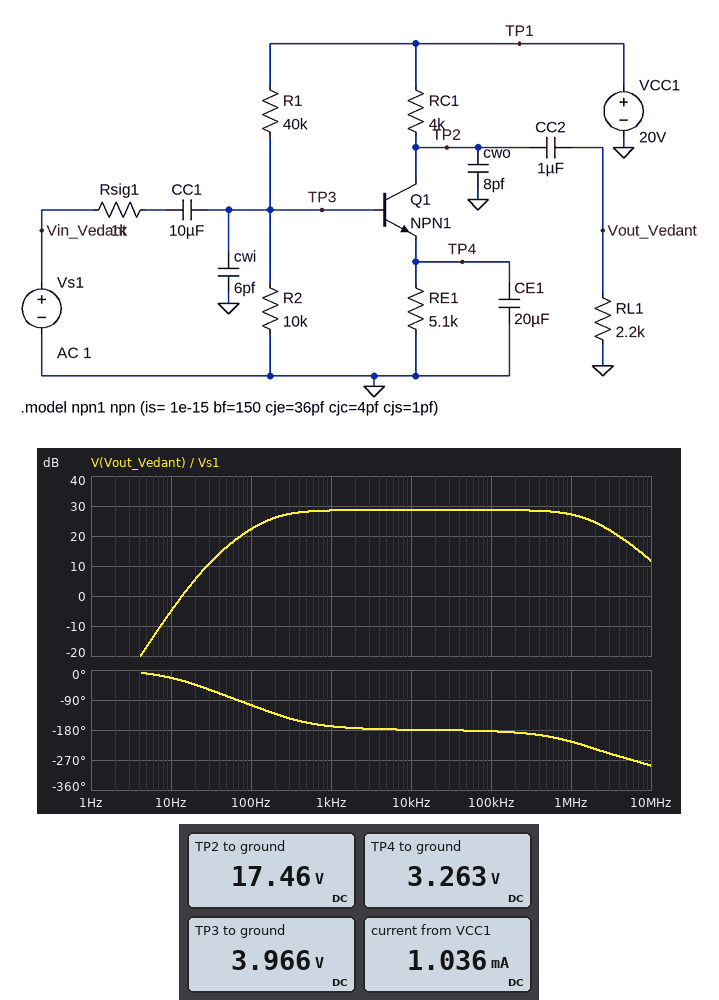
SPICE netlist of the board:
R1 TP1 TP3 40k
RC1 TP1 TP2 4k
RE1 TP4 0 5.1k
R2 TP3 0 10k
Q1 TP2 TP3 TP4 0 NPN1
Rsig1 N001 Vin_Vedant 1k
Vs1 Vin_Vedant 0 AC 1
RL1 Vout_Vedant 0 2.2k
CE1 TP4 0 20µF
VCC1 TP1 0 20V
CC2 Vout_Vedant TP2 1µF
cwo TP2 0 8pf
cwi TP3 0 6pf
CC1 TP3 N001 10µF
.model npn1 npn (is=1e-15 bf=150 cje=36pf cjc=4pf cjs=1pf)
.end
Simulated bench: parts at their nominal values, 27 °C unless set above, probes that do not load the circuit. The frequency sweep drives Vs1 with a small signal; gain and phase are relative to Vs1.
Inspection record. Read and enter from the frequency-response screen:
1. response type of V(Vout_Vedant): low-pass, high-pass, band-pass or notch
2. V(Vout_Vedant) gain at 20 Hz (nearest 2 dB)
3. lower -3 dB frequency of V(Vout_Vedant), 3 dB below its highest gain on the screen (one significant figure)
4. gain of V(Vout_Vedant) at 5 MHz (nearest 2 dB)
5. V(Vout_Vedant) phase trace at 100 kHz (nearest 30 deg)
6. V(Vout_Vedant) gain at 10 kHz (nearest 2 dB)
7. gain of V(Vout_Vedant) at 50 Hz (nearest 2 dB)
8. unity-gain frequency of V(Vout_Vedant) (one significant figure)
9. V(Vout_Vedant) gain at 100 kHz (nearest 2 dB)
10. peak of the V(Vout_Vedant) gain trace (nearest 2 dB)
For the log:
band-pass
6 dB
200 Hz
18 dB
-180 deg
28 dB
16 dB
10 Hz
28 dB
28 dB
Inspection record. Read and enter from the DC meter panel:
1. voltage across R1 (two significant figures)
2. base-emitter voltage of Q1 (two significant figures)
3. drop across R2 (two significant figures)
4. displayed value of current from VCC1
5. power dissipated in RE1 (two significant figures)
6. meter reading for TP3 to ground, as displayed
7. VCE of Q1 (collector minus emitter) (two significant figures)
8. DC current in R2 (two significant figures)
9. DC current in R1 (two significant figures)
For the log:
16 V
700 mV
4.0 V
1.036 mA
2.1 mW
3.966 V
14 V
400 µA
400 µA
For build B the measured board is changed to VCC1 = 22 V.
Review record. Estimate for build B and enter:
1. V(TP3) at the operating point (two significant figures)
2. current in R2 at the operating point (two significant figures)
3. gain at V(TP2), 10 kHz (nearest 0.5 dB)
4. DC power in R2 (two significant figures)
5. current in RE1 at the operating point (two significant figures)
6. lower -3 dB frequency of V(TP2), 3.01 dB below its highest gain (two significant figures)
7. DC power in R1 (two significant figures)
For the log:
4.4 V
440 µA
29.5 dB
1.9 mW
720 µA
170 Hz
7.8 mW
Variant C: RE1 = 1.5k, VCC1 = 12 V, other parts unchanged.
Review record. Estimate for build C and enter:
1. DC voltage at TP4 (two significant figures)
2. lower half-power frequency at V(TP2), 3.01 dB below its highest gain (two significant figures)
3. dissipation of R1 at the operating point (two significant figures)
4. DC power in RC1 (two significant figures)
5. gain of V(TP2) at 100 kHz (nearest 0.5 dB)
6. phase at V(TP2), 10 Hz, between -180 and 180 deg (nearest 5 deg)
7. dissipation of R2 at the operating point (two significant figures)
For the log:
1.6 V
260 Hz
2.3 mW
4.6 mW
32.5 dB
-125 deg
550 µW
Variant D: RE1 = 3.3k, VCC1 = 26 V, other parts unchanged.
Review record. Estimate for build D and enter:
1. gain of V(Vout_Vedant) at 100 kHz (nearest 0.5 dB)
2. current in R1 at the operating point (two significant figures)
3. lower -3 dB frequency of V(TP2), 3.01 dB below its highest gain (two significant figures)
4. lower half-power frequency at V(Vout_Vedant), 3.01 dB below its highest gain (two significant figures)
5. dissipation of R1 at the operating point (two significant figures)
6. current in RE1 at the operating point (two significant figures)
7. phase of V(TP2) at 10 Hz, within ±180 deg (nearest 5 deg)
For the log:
34.0 dB
520 µA
310 Hz
320 Hz
11 mW
1.3 mA
-110 deg
